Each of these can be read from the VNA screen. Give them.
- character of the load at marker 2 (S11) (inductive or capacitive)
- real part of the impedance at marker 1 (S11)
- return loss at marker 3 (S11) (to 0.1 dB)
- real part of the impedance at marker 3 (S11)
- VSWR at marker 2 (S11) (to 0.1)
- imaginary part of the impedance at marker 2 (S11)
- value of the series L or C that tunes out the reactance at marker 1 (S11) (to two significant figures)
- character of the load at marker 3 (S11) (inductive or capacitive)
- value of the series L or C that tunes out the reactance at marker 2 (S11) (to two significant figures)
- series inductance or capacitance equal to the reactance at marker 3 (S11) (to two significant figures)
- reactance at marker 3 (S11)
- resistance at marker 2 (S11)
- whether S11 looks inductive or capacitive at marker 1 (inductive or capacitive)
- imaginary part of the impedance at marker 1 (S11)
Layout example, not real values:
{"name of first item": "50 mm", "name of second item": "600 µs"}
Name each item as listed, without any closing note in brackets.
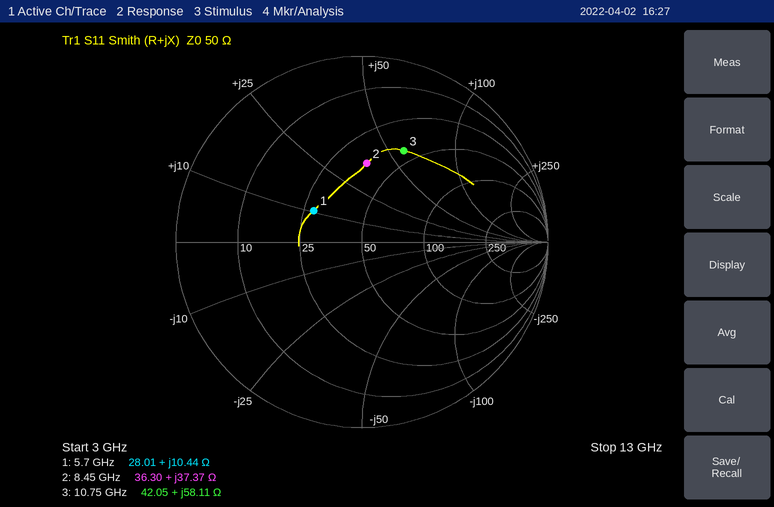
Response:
{"character of the load at marker 2 (S11)": "inductive", "real part of the impedance at marker 1": "28.01 Ω", "return loss at marker 3 (S11)": "5.4 dB", "real part of the impedance at marker 3": "42.05 Ω", "VSWR at marker 2 (S11)": "2.5", "imaginary part of the impedance at marker 2": "+37.37 Ω", "value of the series L or C that tunes out the reactance at marker 1 (S11)": "2.7 pF", "character of the load at marker 3 (S11)": "inductive", "value of the series L or C that tunes out the reactance at marker 2 (S11)": "500 fF", "series inductance or capacitance equal to the reactance at marker 3 (S11)": "860 pH", "reactance at marker 3": "+58.11 Ω", "resistance at marker 2": "36.30 Ω", "whether S11 looks inductive or capacitive at marker 1": "inductive", "imaginary part of the impedance at marker 1": "+10.44 Ω"}
